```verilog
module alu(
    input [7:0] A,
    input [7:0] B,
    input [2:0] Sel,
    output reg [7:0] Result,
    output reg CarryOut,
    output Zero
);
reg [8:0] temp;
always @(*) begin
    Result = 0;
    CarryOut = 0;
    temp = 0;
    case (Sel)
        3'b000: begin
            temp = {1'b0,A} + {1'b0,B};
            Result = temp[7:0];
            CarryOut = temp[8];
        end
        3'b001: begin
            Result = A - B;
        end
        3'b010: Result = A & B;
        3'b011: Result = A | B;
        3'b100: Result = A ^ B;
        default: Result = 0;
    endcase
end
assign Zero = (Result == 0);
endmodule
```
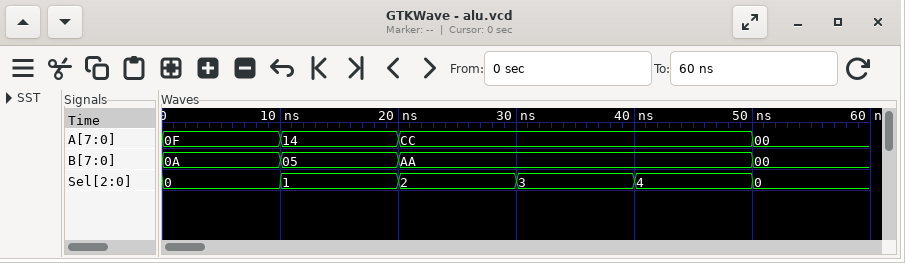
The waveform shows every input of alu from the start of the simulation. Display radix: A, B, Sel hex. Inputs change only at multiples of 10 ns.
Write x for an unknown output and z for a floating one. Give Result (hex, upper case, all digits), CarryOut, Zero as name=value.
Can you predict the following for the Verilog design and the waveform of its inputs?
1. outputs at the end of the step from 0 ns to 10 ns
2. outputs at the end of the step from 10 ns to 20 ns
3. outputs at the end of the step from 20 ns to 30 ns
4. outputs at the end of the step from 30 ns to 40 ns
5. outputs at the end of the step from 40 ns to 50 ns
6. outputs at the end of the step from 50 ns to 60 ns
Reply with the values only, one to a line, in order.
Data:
Result=19, CarryOut=0, Zero=0
Result=0F, CarryOut=0, Zero=0
Result=88, CarryOut=0, Zero=0
Result=EE, CarryOut=0, Zero=0
Result=66, CarryOut=0, Zero=0
Result=00, CarryOut=0, Zero=1
